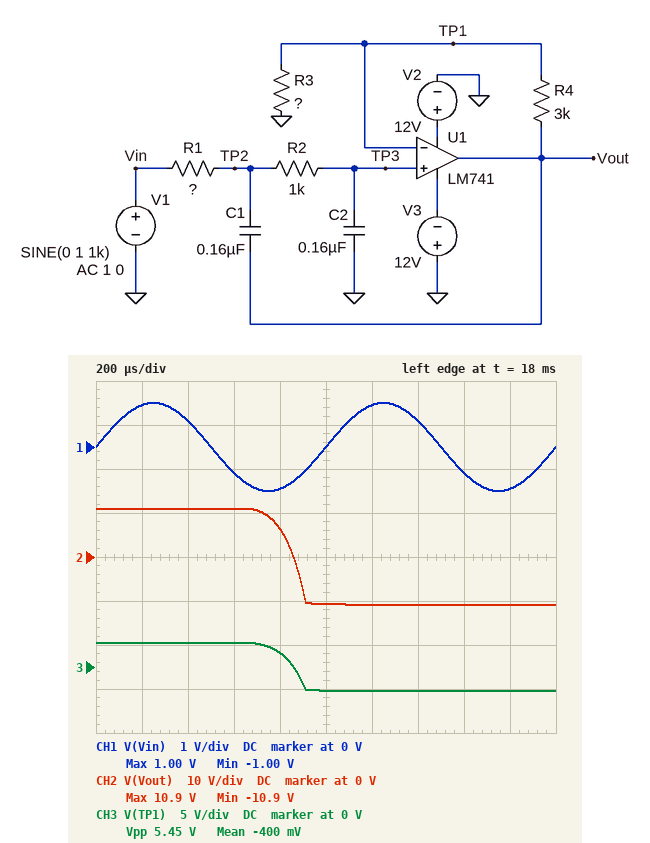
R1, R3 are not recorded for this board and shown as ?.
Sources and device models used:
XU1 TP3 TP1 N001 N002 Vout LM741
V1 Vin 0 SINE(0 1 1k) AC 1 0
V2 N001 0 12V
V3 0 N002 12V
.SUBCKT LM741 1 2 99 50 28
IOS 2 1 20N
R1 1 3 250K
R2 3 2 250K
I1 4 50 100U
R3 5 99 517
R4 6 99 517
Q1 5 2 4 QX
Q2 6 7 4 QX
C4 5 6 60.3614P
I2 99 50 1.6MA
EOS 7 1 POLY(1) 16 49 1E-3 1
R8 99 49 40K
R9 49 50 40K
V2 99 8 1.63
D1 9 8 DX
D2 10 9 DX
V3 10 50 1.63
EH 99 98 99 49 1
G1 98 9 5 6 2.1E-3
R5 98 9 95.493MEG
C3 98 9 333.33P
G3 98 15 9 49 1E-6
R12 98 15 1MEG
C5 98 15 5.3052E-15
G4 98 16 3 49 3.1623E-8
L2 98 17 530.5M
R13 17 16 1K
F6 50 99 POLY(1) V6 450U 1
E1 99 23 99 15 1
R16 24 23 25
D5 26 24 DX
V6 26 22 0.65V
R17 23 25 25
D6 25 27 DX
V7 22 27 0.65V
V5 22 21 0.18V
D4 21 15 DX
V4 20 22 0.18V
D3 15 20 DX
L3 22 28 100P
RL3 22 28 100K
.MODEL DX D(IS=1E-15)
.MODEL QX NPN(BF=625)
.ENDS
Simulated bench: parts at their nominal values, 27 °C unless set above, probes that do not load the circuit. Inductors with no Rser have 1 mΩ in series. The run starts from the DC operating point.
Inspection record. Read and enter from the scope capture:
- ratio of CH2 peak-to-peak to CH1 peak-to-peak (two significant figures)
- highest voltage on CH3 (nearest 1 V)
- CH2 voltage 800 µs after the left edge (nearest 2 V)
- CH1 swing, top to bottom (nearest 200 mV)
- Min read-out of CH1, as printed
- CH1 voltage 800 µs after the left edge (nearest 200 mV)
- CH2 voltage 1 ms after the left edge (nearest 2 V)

11
3 V
6 V
2.0 V
-1.00 V
-1.0 V
-10 V
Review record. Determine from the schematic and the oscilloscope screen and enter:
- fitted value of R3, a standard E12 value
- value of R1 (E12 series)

1 kΩ
3.3 kΩ
